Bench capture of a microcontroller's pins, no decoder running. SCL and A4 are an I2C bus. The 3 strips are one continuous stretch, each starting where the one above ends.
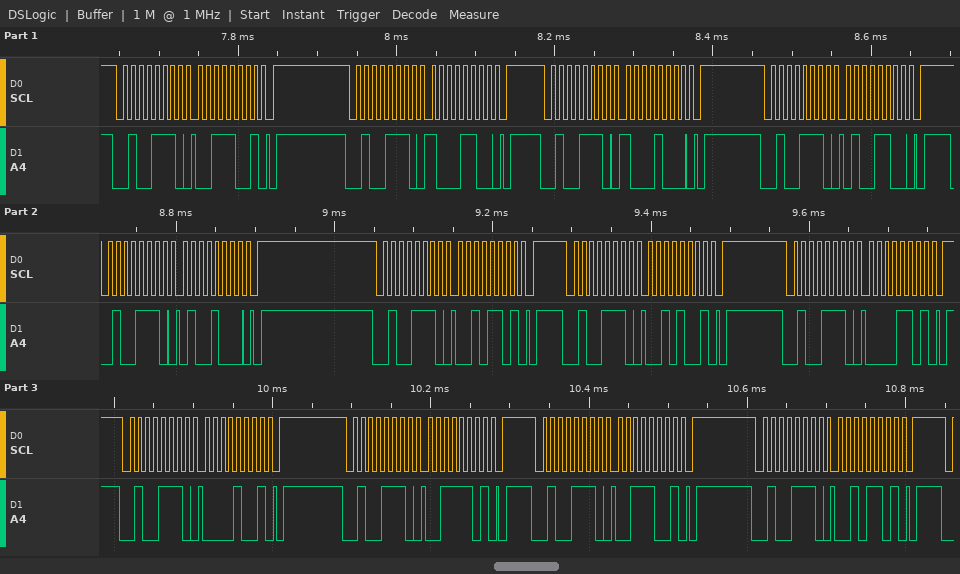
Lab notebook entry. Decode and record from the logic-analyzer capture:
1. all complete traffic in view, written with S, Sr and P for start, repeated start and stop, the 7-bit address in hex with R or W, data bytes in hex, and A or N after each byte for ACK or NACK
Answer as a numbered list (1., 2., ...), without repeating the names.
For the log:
1. S 27W A 39 A P S 27W A 8C A P S 27W A 88 A P S 27W A 4C A P S 27W A 48 A P S 27W A 2D A P S 27W A 29 A P S 27W A 0D A P S 27W A 09 A P S 27W A 3D A P S 27W A 39 A P S 27W A 2D A P
